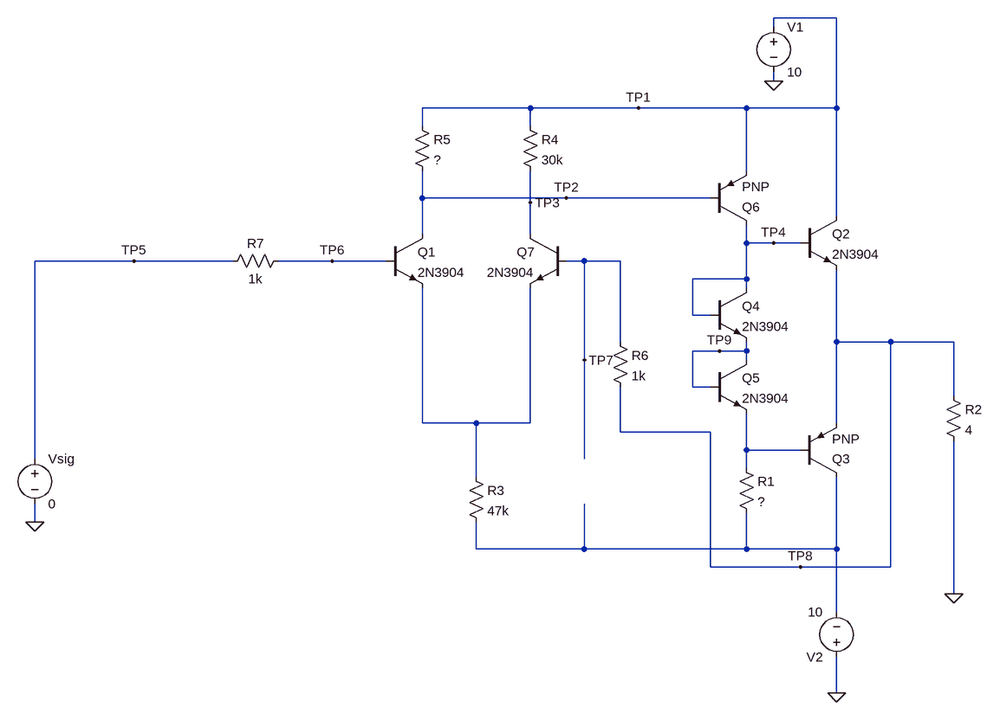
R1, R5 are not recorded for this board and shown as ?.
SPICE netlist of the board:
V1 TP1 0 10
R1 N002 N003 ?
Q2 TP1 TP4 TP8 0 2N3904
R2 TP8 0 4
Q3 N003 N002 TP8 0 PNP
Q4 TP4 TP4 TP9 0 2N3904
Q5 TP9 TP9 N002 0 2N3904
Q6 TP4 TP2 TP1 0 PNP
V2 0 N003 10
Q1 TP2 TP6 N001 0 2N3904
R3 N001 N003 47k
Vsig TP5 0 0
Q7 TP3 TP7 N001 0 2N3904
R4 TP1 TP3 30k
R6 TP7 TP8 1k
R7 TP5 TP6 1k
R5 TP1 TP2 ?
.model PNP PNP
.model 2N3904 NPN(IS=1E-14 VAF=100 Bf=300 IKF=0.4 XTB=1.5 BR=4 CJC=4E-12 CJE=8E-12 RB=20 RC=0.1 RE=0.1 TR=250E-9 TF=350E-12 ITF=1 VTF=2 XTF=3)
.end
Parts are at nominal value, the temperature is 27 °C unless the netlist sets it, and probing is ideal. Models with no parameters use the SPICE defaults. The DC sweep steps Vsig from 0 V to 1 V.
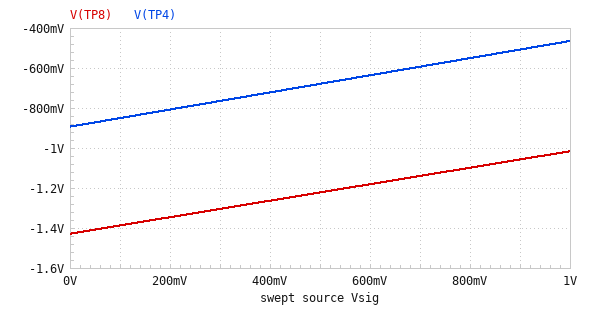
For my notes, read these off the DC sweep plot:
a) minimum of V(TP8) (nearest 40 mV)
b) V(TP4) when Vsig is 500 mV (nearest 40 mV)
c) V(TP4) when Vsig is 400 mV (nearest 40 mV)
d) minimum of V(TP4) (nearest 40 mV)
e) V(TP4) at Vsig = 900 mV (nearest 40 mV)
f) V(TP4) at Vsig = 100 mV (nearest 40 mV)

-1.44 V
-680 mV
-720 mV
-880 mV
-520 mV
-840 mV
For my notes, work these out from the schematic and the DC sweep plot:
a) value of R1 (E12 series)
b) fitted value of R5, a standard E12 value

390 Ω
22 kΩ
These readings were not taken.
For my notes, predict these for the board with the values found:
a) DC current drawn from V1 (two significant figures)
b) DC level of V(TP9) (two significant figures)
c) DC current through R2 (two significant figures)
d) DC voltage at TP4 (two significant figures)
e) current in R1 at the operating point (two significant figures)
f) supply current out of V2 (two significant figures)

16 mA
-1.6 V
360 mA
-890 mV
20 mA
370 mA
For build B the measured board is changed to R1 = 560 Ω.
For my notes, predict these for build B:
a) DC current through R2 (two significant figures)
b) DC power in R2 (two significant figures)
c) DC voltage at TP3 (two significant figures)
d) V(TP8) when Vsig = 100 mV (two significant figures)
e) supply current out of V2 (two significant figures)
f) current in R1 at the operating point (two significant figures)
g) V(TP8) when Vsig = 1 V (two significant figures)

29 mA
3.3 mW
9.9 V
-41 mV
45 mA
16 mA
530 mV
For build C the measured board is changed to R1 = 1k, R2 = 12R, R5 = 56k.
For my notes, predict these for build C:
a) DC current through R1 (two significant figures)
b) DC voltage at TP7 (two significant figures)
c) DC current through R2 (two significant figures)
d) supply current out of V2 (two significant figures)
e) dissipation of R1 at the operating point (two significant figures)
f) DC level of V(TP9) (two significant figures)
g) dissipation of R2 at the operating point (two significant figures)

9.2 mA
-3.6 mV
280 µA
11 mA
85 mW
-67 mV
920 nW
